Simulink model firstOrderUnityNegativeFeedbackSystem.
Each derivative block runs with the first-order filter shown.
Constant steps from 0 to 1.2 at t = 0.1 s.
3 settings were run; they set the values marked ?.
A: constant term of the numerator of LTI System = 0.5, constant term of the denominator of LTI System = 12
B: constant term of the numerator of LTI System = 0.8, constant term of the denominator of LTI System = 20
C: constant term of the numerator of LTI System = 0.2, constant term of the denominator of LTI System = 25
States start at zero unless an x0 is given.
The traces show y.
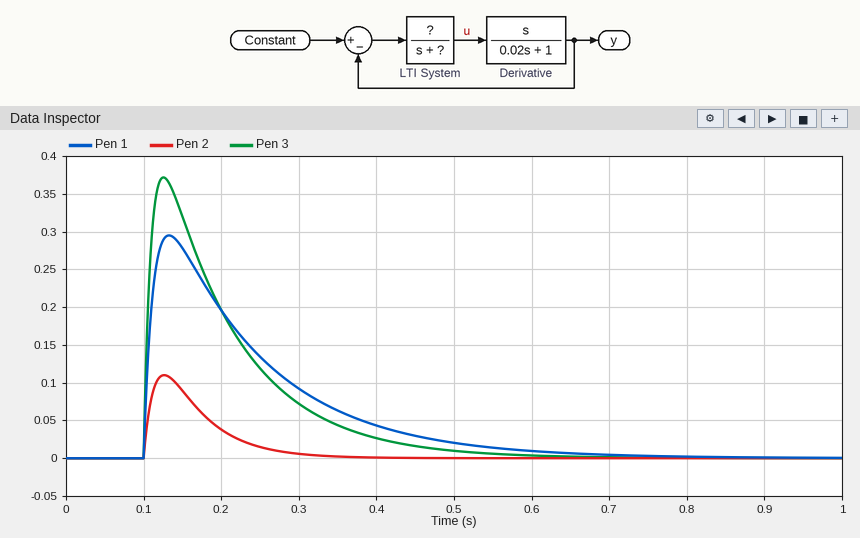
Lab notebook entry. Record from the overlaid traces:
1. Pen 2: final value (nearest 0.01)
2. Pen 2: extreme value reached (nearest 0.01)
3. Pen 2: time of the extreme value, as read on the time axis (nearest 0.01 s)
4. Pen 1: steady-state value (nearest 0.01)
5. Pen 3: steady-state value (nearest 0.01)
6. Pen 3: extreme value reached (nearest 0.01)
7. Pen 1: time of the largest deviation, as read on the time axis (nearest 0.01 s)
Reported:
0.00
0.11
0.13 s
0.00
0.00
0.37
0.13 s
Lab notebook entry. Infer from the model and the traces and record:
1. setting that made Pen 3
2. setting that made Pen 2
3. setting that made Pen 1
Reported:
B
C
A
